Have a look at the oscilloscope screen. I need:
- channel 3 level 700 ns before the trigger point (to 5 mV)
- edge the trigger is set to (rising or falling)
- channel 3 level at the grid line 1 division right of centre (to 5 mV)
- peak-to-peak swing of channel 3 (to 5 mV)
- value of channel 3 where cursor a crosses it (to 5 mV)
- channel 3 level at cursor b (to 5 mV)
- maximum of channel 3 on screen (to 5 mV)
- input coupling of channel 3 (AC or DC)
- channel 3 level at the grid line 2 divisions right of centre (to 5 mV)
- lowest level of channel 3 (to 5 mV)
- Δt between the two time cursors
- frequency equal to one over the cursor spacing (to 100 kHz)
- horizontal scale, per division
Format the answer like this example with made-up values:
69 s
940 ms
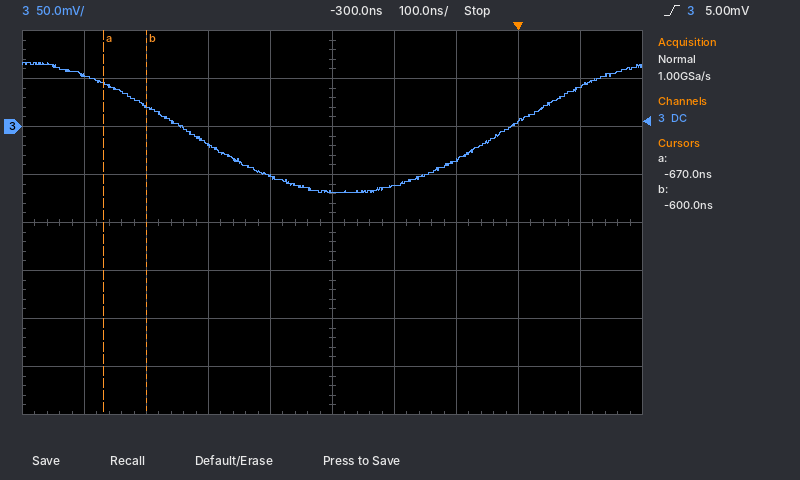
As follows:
55 mV
rising
-60 mV
135 mV
45 mV
20 mV
65 mV
DC
-35 mV
-70 mV
70 ns
14.3 MHz
100 ns
